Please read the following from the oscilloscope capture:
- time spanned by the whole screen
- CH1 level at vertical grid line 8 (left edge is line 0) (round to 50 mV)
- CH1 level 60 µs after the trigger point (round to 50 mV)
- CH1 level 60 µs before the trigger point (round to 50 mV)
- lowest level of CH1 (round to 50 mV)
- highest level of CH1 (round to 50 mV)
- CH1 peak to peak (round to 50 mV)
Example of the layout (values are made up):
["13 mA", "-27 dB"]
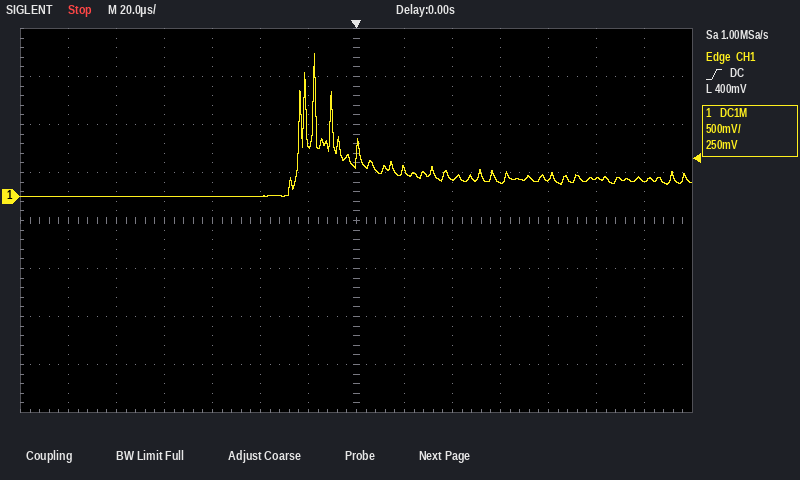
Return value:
["280 µs", "300 mV", "150 mV", "0 mV", "0 mV", "1.50 V", "1.50 V"]
